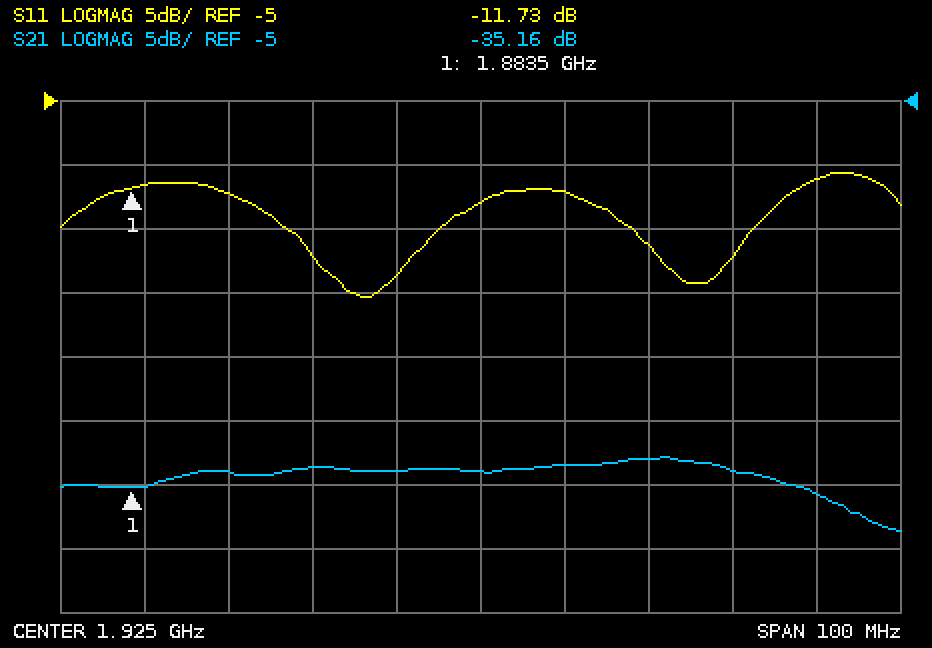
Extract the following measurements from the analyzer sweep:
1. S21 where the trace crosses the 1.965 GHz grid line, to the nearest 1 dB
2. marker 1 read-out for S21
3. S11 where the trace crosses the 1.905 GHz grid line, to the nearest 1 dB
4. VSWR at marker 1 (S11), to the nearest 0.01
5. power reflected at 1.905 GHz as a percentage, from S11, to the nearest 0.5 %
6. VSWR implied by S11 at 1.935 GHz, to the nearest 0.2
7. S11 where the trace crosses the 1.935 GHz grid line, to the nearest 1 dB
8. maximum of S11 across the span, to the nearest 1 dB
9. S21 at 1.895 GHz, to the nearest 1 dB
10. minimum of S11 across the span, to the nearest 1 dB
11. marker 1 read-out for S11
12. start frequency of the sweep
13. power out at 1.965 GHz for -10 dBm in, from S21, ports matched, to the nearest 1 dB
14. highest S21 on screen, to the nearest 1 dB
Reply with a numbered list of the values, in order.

1. -36 dB
2. -35.16 dB
3. -17 dB
4. 1.70
5. 2.0 %
6. 1.6
7. -12 dB
8. -11 dB
9. -34 dB
10. -20 dB
11. -11.73 dB
12. 1.875 GHz
13. -46 dBm
14. -33 dB
